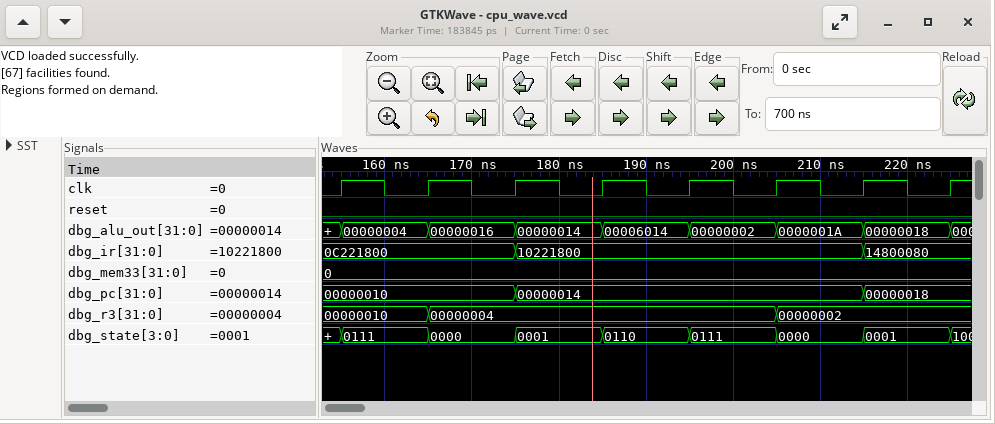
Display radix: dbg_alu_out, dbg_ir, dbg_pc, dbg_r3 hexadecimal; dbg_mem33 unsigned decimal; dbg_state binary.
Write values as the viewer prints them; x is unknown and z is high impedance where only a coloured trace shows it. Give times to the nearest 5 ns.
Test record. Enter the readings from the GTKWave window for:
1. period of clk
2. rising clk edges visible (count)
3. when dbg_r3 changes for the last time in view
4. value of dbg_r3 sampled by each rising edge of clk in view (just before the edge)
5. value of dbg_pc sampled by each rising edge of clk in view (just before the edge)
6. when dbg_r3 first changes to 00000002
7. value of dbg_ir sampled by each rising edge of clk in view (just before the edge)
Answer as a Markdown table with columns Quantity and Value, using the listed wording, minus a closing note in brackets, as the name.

| Quantity | Value |
|---|---|
| period of clk | 10 ns |
| rising clk edges visible | 8 |
| when dbg_r3 changes for the last time in view | 205 ns |
| value of dbg_r3 sampled by each rising edge of clk in view | 00000010, 00000010, 00000004, 00000004, 00000004, 00000004, 00000002, 00000002 |
| value of dbg_pc sampled by each rising edge of clk in view | 00000010, 00000010, 00000010, 00000014, 00000014, 00000014, 00000014, 00000018 |
| when dbg_r3 first changes to 00000002 | 205 ns |
| value of dbg_ir sampled by each rising edge of clk in view | 0C221800, 0C221800, 0C221800, 10221800, 10221800, 10221800, 10221800, 14800080 |
